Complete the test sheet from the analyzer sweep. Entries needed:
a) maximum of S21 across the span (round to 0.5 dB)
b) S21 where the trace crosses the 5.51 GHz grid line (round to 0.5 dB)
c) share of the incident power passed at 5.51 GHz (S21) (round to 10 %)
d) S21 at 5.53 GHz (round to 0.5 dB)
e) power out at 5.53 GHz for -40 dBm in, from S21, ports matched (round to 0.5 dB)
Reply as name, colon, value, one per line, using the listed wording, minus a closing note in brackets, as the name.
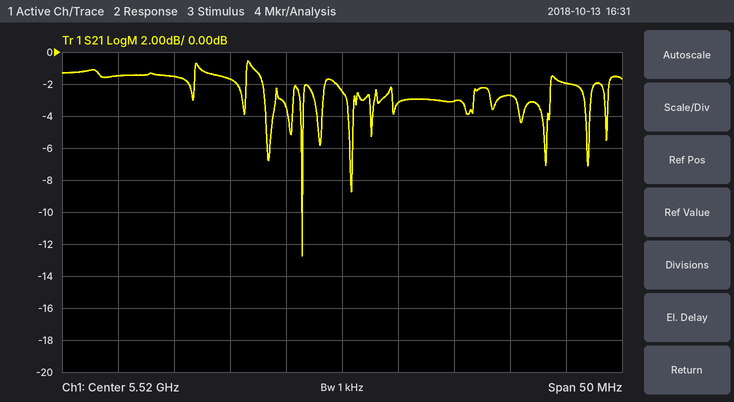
maximum of S21 across the span: -0.5 dB
S21 where the trace crosses the 5.51 GHz grid line: -1.5 dB
share of the incident power passed at 5.51 GHz (S21): 70 %
S21 at 5.53 GHz: -3.0 dB
power out at 5.53 GHz for -40 dBm in, from S21, ports matched: -43.0 dBm
